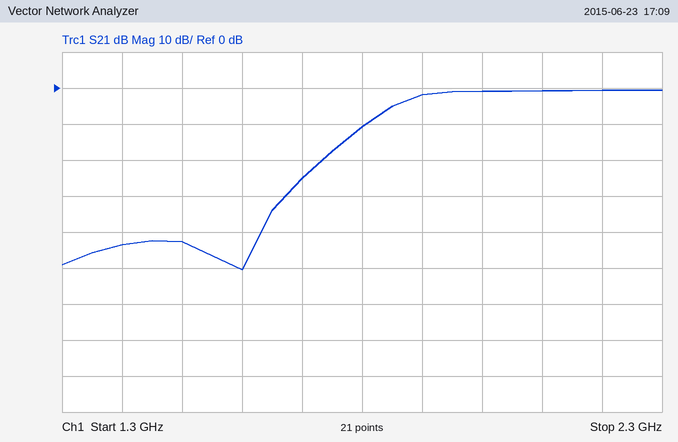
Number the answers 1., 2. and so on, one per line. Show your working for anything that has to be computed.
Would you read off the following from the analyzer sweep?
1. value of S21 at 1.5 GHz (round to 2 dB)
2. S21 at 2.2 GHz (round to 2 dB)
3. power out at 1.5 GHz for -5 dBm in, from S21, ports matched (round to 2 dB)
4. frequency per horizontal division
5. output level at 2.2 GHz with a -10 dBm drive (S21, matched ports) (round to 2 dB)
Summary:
1. -42 dB
2. 0 dB
3. -5 dBm + (-42 dB) = -48 dBm
4. 100 MHz
5. -10 dBm + (0 dB) = -10 dBm
